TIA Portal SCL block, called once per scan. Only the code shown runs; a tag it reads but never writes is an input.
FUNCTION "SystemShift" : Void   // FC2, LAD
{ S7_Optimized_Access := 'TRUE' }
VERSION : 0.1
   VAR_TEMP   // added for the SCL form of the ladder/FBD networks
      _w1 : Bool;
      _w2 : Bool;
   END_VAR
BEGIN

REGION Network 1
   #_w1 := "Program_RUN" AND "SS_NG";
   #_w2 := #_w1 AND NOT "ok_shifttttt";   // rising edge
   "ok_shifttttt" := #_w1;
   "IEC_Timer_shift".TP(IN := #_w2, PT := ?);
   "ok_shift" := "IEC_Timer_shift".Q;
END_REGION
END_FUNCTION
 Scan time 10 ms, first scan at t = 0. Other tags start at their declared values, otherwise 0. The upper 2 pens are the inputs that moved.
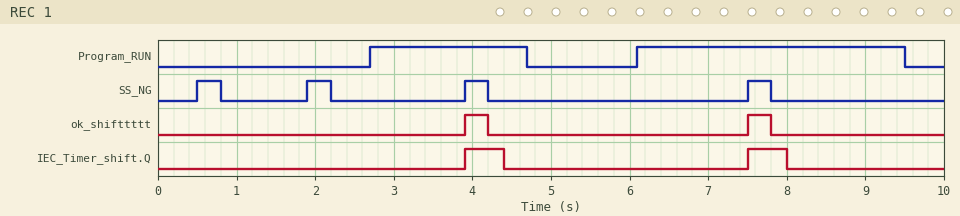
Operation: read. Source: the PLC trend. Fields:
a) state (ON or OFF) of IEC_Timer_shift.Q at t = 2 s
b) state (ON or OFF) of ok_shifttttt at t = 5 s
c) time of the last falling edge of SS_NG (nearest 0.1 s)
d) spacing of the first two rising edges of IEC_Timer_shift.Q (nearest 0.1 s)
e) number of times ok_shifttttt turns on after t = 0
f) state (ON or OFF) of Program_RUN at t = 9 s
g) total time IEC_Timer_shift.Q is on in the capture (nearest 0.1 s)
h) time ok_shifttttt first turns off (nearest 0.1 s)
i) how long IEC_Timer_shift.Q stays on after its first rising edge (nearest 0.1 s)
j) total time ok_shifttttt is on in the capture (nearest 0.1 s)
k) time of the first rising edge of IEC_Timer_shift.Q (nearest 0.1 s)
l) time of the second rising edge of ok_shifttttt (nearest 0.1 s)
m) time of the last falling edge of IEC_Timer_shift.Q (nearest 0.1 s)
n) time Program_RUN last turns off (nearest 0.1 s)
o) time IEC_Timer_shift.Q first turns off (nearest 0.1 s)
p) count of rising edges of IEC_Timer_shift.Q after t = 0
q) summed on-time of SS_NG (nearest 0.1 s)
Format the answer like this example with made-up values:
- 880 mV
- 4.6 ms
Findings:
- OFF
- OFF
- 7.8 s
- 3.6 s
- 2
- ON
- 1.0 s
- 4.2 s
- 0.5 s
- 0.6 s
- 3.9 s
- 7.5 s
- 8.0 s
- 9.5 s
- 4.4 s
- 2
- 1.2 s
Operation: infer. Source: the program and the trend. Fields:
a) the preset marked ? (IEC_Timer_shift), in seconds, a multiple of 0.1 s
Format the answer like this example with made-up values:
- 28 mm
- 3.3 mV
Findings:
- 0.5 s
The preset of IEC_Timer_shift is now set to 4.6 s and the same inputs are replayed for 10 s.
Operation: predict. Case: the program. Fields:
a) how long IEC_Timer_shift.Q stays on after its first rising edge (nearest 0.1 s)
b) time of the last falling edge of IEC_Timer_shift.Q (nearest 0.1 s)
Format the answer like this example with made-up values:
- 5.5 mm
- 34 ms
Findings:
- 4.6 s
- 8.5 s
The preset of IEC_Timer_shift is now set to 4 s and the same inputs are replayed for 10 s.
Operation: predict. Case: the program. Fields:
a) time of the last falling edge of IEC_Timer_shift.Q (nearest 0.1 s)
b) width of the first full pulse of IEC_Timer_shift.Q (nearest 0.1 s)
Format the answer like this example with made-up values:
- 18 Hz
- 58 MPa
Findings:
- 7.9 s
- 4.0 s
